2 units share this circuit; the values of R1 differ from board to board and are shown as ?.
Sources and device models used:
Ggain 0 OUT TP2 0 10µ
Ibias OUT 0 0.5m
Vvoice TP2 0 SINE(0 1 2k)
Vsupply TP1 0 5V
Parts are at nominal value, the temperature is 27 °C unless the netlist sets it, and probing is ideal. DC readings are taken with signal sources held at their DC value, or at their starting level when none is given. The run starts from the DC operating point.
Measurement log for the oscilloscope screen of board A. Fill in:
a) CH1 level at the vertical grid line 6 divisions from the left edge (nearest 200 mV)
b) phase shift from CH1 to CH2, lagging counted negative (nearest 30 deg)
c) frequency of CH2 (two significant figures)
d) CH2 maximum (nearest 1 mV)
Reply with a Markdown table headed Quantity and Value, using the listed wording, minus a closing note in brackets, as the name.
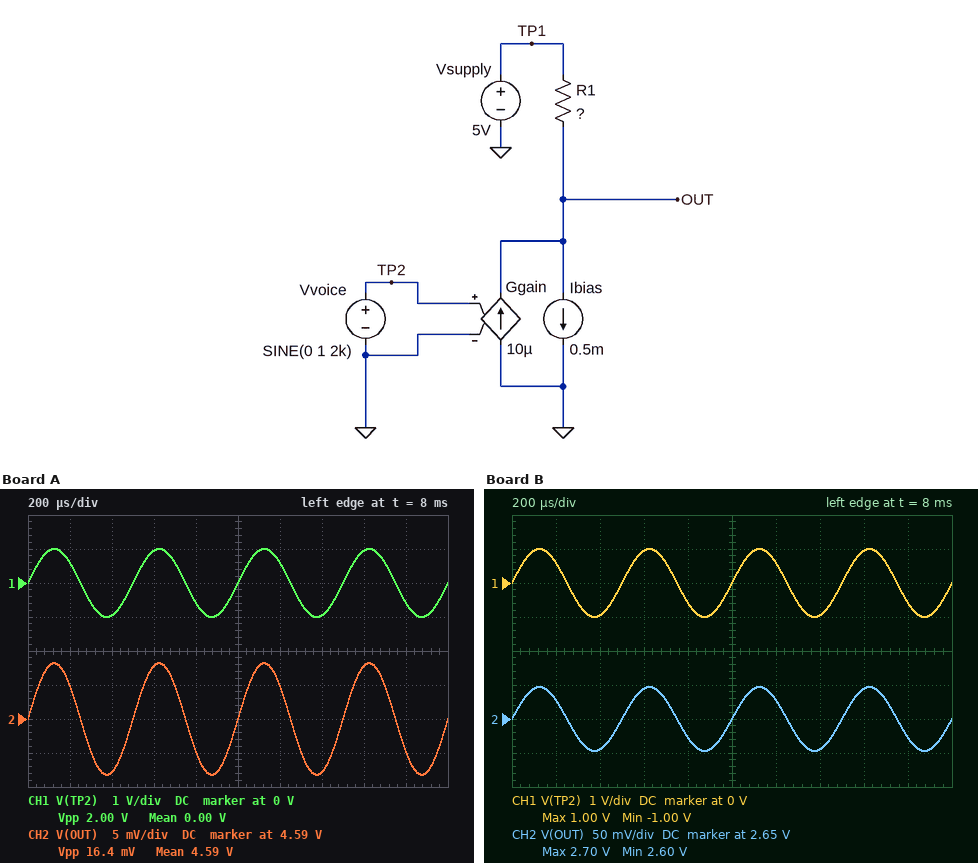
| Quantity | Value |
|---|---|
| CH1 level at the vertical grid line 6 divisions from the left edge | 600 mV |
| phase shift from CH1 to CH2, lagging counted negative | 0 deg |
| frequency of CH2 | 2.0 kHz |
| CH2 maximum | 4.598 V |
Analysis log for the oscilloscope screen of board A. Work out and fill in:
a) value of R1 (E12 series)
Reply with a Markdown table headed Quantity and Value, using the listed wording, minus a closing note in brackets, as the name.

| Quantity | Value |
|---|---|
| value of R1 | 820 Ω |
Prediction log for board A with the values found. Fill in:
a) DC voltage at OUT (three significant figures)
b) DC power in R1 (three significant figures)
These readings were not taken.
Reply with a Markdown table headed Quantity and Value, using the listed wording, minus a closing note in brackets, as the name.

| Quantity | Value |
|---|---|
| DC voltage at OUT | 4.59 V |
| DC power in R1 | 205 µW |
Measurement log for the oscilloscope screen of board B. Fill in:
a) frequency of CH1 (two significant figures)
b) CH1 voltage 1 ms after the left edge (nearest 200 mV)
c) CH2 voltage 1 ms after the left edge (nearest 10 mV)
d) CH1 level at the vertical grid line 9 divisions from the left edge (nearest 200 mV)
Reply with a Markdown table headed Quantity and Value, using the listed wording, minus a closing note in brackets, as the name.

| Quantity | Value |
|---|---|
| frequency of CH1 | 2.0 kHz |
| CH1 voltage 1 ms after the left edge | 0 V |
| CH2 voltage 1 ms after the left edge | 2.65 V |
| CH1 level at the vertical grid line 9 divisions from the left edge | -600 mV |
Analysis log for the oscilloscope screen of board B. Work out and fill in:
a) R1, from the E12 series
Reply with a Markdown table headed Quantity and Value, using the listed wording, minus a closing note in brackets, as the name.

| Quantity | Value |
|---|---|
| R1, from the E12 series | 4.7 kΩ |
